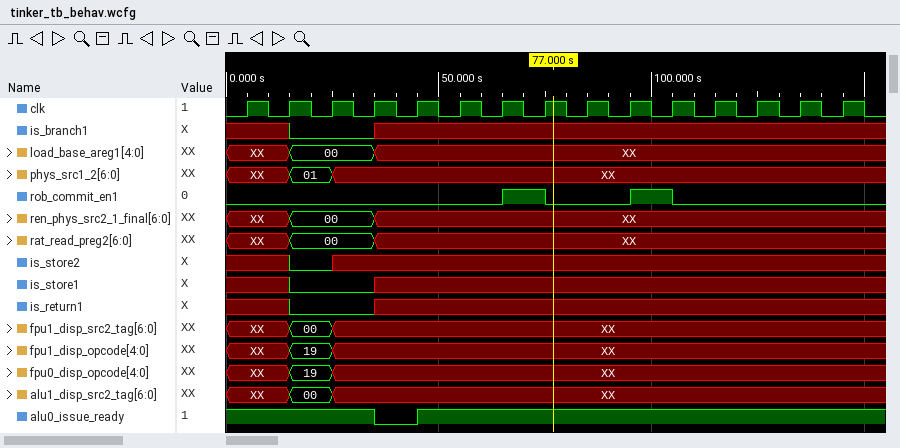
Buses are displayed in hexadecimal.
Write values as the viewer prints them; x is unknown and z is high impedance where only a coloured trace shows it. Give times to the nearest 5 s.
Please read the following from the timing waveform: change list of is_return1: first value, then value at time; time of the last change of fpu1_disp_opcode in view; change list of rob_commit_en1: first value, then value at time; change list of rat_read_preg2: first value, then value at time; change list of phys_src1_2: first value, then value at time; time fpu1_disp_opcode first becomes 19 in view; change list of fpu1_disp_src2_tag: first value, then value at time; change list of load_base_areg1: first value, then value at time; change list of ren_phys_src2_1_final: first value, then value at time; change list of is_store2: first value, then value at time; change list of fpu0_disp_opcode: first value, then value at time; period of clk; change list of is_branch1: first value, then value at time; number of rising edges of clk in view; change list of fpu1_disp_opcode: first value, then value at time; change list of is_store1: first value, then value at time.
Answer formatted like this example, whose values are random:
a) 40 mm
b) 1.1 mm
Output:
a) x, 0 at 15 s, x at 35 s
b) 25 s
c) 0, 1 at 65 s, 0 at 75 s, 1 at 95 s, 0 at 105 s
d) XX, 00 at 15 s, XX at 35 s
e) XX, 01 at 15 s, XX at 25 s
f) 15 s
g) XX, 00 at 15 s, XX at 25 s
h) XX, 00 at 15 s, XX at 35 s
i) XX, 00 at 15 s, XX at 35 s
j) x, 0 at 15 s, x at 25 s
k) XX, 19 at 15 s, XX at 25 s
l) 10 s
m) x, 0 at 15 s, x at 35 s
n) 15
o) XX, 19 at 15 s, XX at 25 s
p) x, 0 at 15 s, x at 35 s
